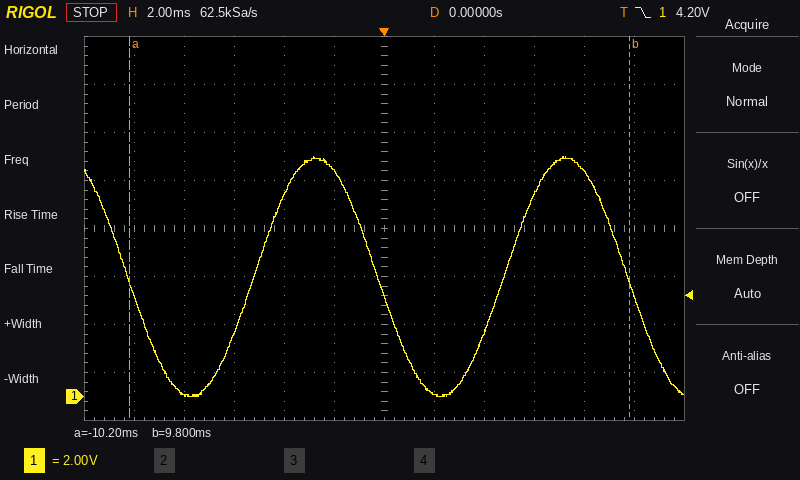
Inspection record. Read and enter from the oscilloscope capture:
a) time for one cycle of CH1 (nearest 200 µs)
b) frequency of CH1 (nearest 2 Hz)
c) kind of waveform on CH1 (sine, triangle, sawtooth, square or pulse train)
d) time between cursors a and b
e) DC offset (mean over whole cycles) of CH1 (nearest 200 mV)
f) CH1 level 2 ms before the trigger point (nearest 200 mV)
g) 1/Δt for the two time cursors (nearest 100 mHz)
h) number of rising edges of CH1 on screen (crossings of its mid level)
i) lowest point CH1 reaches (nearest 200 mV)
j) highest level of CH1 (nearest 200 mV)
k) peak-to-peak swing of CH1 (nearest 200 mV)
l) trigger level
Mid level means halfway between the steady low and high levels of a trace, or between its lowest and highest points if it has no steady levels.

10.0 ms
100 Hz
sine
20.0 ms
5.0 V
9.4 V
50.0 Hz
2
0.0 V
10.0 V
10.0 V
4.20 V
